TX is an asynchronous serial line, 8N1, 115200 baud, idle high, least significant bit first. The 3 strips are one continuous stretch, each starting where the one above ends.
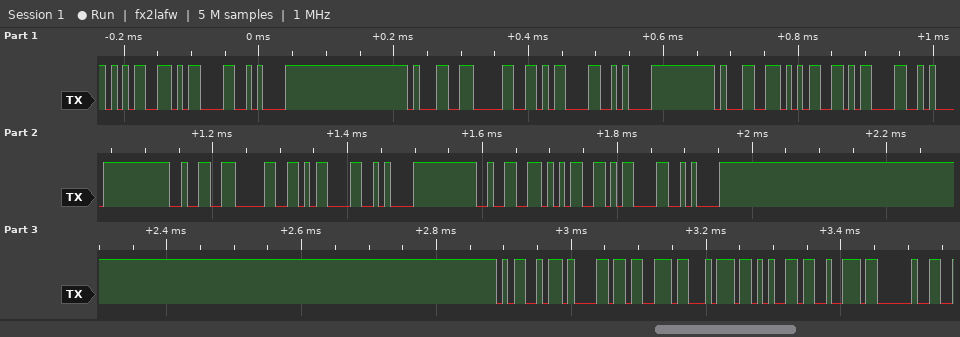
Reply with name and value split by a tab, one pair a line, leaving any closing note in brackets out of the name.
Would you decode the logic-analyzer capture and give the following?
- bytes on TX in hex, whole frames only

bytes on TX in hex, whole frames only	35 0D 0A 31 30 0D 0A 31 35 0D 0A 32 30 0D 0A 32 35 0D 0A 4D 61 73 74 65 72 20
